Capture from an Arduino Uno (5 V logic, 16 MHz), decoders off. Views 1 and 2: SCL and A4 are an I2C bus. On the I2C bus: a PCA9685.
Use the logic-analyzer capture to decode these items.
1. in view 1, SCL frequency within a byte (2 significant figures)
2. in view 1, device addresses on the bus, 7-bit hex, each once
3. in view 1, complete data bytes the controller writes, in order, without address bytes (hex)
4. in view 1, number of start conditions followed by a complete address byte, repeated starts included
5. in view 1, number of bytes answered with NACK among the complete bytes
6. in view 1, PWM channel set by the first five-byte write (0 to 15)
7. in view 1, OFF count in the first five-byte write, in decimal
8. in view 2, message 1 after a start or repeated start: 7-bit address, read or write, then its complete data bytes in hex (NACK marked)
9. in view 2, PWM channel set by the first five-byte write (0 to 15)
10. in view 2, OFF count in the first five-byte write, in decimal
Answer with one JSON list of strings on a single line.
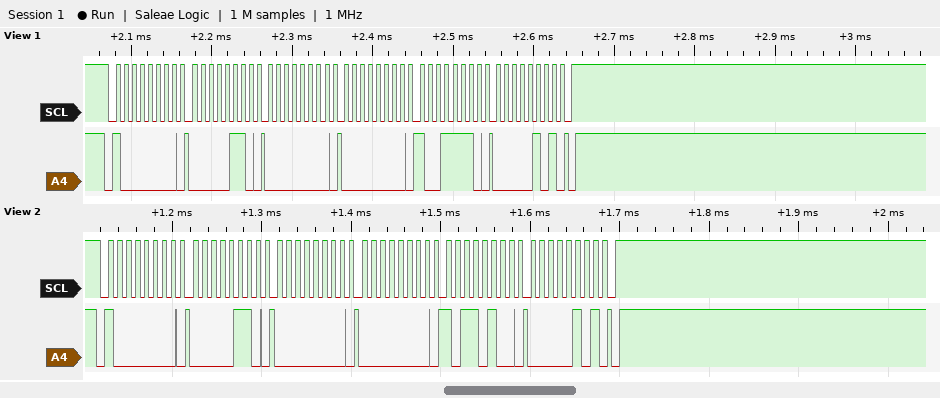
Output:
["100 kHz", "0x40", "06 00 00 9E 05", "1", "0", "0", "1438", "0x40 write: 06 00 00 B4 05", "0", "1460"]
